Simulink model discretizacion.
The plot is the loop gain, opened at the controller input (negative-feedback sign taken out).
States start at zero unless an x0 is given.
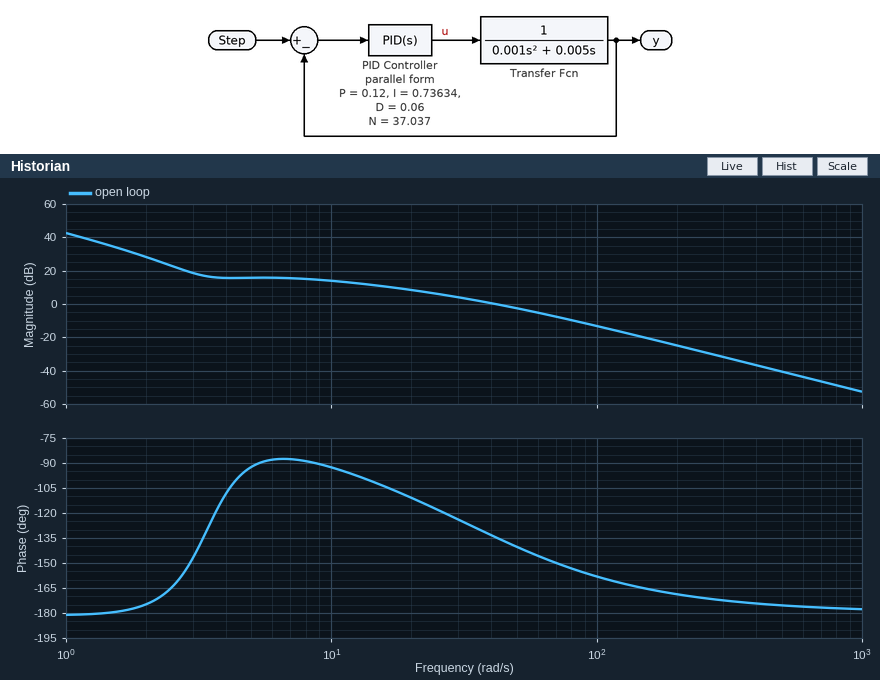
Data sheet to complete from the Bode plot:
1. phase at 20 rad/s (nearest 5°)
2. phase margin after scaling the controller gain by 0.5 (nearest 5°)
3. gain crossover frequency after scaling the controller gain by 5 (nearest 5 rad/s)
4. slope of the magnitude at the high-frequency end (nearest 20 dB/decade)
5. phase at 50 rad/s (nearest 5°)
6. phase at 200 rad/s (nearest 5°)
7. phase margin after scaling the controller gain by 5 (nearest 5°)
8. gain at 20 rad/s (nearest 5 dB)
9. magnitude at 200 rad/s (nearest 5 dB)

-110°
60°
105 rad/s
-40 dB/decade
-140°
-170°
20°
10 dB
-25 dB
